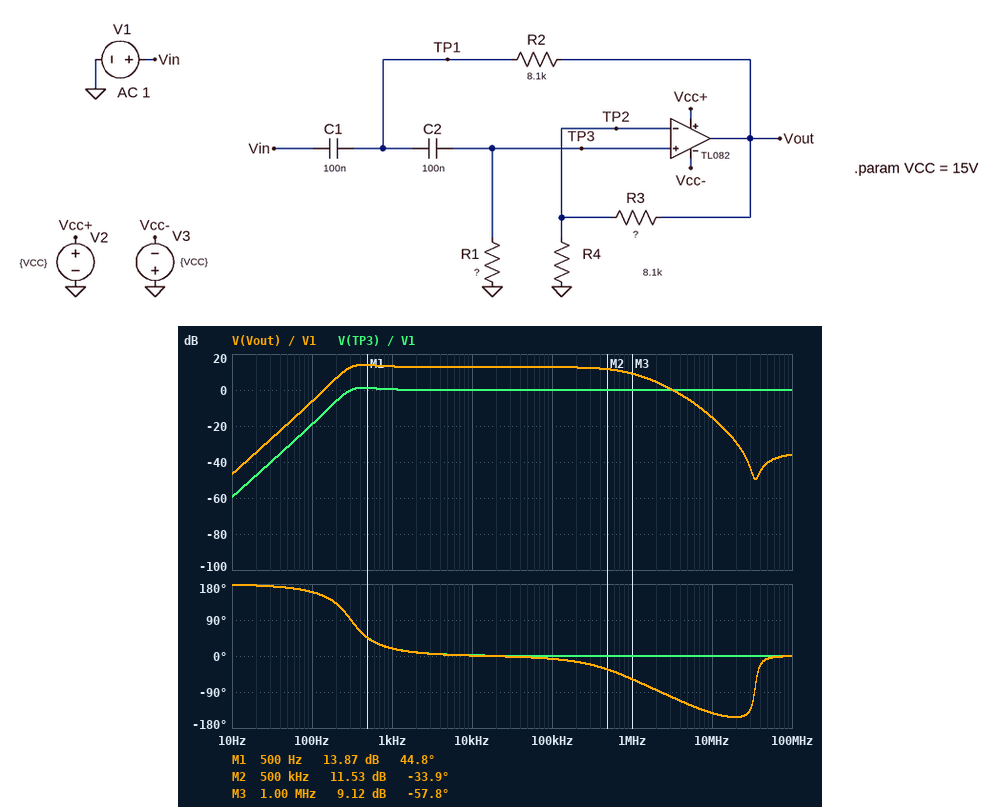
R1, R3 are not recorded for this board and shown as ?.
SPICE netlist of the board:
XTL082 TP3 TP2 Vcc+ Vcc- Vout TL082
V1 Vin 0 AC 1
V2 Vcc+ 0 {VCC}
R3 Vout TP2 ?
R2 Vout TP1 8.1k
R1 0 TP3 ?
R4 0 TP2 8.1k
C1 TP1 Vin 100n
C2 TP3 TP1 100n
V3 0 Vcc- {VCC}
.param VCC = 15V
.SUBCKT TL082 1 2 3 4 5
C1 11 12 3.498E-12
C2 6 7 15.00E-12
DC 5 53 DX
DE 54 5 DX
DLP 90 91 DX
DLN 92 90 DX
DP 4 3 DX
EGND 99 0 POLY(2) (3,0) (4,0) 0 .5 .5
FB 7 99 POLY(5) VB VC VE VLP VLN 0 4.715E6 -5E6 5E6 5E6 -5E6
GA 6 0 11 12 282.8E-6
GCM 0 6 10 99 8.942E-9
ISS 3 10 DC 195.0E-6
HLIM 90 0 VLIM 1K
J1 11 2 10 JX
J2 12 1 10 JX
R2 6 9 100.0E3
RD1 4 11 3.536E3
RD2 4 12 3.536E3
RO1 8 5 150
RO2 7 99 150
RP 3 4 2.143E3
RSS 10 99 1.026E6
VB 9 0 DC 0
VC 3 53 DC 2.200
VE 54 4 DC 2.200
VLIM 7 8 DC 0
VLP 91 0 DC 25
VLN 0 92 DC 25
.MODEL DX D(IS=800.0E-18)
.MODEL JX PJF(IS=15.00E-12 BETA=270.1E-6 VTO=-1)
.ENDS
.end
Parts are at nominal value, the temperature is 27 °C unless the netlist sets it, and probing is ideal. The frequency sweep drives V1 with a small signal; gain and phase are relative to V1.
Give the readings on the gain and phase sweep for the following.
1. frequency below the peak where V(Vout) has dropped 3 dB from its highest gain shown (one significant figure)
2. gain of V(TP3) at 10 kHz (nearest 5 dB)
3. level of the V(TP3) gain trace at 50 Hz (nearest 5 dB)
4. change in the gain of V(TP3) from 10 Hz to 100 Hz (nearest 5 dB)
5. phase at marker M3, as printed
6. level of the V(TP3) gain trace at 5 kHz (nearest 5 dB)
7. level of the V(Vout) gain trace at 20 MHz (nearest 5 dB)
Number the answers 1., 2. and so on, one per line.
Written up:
1. 300 Hz
2. 0 dB
3. -30 dB
4. 40 dB
5. -57.8 deg
6. 0 dB
7. -30 dB
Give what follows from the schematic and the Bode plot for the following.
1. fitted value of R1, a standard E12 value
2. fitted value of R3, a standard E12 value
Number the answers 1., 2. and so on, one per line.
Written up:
1. 3.3 kΩ
2. 27 kΩ
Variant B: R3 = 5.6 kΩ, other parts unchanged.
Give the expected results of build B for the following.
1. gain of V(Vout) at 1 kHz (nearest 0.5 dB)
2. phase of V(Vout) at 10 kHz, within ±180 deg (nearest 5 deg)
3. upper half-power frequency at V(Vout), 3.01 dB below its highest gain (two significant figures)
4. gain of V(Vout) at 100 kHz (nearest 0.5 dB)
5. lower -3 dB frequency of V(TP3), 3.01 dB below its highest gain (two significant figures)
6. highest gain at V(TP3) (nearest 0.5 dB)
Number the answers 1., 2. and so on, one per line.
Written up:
1. 3.0 dB
2. 5 deg
3. 2.6 MHz
4. 4.5 dB
5. 720 Hz
6. 0 dB
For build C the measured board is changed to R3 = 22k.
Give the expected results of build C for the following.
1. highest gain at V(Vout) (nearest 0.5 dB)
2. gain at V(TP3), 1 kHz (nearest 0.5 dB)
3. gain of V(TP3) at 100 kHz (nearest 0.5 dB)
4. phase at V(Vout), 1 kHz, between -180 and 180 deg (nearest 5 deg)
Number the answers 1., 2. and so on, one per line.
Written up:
1. 11.5 dB
2. 0 dB
3. 0 dB
4. 25 deg
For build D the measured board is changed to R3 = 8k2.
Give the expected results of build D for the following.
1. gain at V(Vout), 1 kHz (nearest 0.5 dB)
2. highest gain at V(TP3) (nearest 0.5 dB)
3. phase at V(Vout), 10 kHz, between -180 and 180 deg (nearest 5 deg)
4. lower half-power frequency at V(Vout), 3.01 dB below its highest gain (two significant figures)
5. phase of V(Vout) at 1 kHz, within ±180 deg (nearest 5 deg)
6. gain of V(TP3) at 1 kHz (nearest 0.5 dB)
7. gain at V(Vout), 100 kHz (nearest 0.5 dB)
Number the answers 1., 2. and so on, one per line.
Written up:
1. 4.5 dB
2. 0 dB
3. 5 deg
4. 650 Hz
5. 40 deg
6. -1.5 dB
7. 6.0 dB
